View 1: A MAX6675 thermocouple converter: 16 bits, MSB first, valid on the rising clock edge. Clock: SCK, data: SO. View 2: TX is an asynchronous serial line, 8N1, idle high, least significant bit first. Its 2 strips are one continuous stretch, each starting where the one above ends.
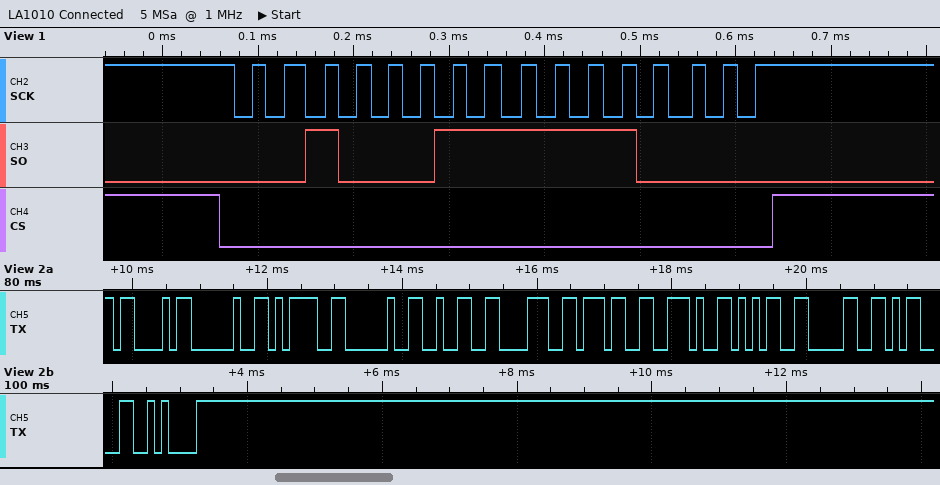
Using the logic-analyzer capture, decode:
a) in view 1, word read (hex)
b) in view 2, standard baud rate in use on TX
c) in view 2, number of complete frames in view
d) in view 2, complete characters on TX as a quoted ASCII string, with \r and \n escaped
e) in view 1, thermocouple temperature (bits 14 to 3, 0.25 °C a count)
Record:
0x23F0
9600 baud
12
"C = 287.50\r\n"
287.50 °C
